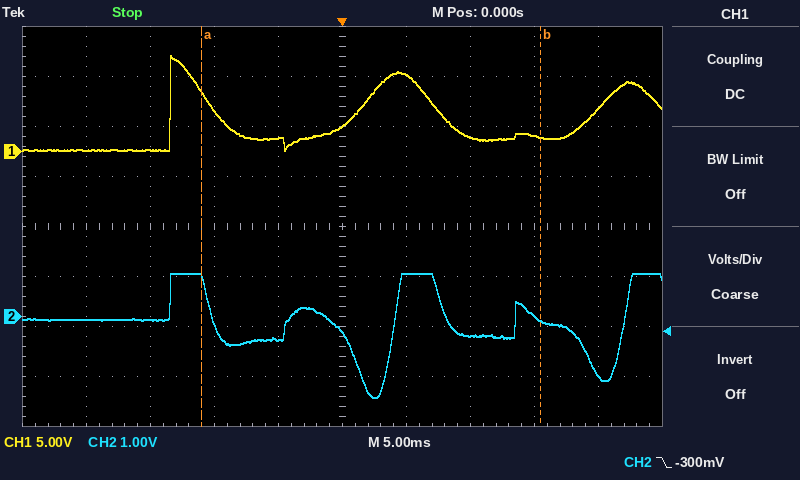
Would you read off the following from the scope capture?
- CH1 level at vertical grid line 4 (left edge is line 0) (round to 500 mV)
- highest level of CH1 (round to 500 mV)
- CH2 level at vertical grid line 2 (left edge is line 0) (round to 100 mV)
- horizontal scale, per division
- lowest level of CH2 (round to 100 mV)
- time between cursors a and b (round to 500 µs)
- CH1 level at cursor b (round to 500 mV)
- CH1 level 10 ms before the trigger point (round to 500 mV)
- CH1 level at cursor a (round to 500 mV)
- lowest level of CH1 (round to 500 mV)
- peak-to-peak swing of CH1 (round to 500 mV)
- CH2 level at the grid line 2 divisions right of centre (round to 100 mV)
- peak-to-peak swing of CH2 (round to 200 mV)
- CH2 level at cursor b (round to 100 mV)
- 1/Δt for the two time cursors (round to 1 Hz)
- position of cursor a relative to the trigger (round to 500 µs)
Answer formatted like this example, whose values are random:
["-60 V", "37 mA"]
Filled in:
["1.5 V", "9.5 V", "-100 mV", "5 ms", "-1.6 V", "26.5 ms", "1.5 V", "4.0 V", "6.0 V", "0.0 V", "9.5 V", "-400 mV", "2.4 V", "-100 mV", "38 Hz", "-11.0 ms"]
